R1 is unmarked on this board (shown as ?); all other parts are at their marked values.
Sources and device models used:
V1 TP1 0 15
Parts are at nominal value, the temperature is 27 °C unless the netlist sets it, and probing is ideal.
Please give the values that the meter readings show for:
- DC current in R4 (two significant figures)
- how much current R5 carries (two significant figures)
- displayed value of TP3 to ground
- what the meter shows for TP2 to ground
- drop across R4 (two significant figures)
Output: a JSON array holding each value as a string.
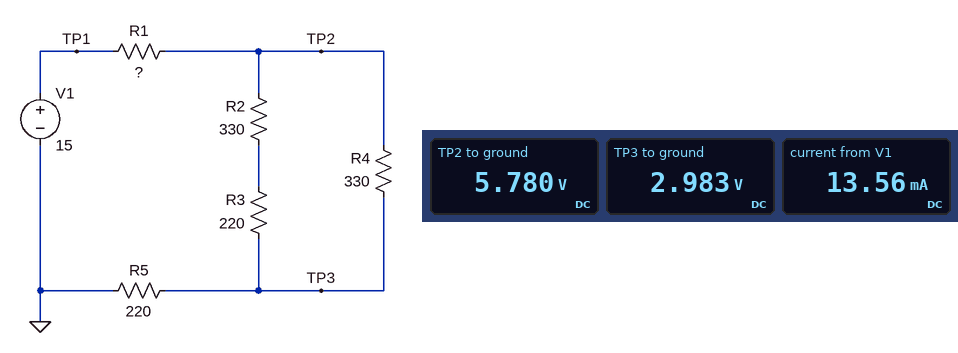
["8.5 mA", "14 mA", "2.983 V", "5.780 V", "2.8 V"]
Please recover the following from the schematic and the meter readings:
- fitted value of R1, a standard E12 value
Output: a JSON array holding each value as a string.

["680 Ω"]
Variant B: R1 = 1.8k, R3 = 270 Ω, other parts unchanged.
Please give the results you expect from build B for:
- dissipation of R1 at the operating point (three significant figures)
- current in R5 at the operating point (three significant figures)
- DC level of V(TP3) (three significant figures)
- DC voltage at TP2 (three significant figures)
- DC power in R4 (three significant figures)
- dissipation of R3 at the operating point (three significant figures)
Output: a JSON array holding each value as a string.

["81.2 mW", "6.72 mA", "1.48 V", "2.91 V", "6.20 mW", "1.53 mW"]
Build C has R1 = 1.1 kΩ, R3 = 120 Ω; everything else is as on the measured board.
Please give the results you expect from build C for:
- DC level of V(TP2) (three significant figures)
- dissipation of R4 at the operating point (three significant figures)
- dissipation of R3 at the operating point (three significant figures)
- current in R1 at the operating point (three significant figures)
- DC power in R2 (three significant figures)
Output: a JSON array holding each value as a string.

["4.08 V", "10.8 mW", "2.12 mW", "9.93 mA", "5.83 mW"]
